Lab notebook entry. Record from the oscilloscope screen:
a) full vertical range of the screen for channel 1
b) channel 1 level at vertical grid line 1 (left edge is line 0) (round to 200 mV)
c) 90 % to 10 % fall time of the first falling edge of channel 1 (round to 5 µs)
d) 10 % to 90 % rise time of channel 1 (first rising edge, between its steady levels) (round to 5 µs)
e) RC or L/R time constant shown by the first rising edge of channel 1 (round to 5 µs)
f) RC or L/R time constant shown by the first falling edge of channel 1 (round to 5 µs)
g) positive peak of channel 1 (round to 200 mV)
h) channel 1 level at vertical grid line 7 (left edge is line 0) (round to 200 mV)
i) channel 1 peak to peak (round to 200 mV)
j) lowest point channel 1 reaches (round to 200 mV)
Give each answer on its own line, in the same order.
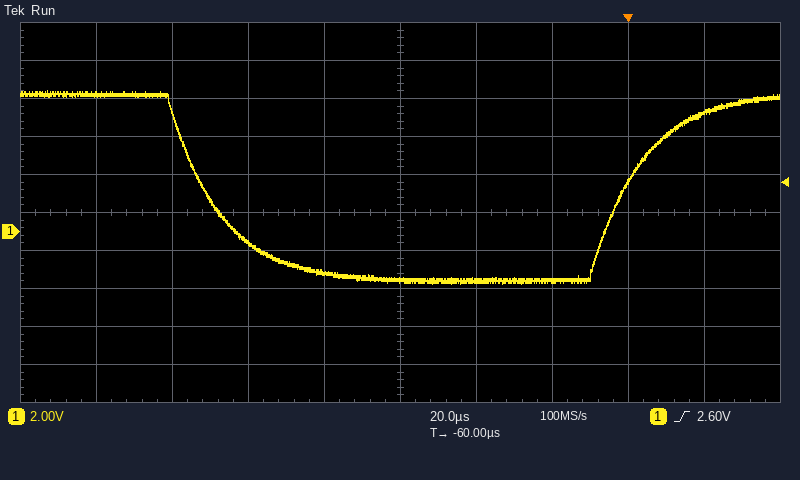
20 V
7.2 V
30 µs
30 µs
15 µs
15 µs
7.4 V
-2.6 V
10.2 V
-2.8 V
